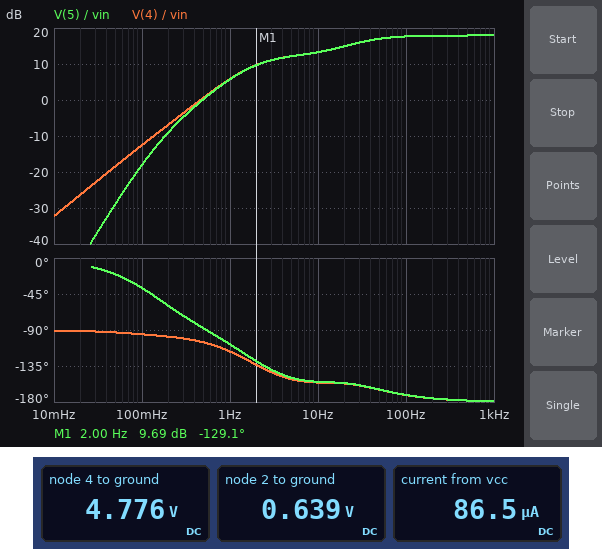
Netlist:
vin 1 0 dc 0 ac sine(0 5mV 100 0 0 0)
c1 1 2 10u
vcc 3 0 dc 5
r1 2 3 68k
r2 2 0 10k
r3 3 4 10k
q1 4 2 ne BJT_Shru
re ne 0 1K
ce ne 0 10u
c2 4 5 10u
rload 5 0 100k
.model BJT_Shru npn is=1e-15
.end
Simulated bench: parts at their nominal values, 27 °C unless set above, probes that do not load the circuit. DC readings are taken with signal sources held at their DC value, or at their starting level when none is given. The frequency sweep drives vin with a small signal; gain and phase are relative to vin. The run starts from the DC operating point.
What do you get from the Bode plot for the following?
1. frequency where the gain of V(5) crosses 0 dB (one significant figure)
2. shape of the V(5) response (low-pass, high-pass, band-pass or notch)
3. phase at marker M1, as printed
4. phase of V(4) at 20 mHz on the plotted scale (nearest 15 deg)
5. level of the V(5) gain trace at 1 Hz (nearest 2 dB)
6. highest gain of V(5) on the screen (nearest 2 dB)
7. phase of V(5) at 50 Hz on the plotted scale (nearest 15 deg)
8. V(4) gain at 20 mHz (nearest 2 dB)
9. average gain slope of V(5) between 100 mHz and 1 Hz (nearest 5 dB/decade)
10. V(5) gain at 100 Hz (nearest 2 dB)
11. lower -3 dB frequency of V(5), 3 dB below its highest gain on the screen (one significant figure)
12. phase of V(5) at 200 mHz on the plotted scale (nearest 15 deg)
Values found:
500 mHz
high-pass
-129.1 deg
-90 deg
6 dB
18 dB
-165 deg
-26 dB
25 dB/decade
18 dB
20 Hz
-60 deg
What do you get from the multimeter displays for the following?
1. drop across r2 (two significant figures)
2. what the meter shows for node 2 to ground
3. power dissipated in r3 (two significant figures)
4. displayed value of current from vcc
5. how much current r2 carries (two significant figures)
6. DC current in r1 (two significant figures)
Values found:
640 mV
0.639 V
5.0 µW
86.5 µA
64 µA
64 µA
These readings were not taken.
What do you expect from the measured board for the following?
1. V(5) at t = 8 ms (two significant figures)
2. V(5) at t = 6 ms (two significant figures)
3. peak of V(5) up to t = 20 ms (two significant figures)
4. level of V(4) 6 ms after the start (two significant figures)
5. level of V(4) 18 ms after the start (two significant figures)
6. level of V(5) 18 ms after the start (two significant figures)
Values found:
33 mV
27 mV
37 mV
4.8 V
4.8 V
33 mV
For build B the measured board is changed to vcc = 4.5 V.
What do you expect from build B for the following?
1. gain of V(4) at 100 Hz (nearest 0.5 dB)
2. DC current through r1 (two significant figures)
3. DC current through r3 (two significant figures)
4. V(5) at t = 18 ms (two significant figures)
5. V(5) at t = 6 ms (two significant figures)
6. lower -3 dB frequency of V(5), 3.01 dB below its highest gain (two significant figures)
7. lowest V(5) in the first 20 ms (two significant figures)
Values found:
3.0 dB
58 µA
4.1 µA
6.3 mV
4.4 mV
2.6 Hz
-7.7 mV
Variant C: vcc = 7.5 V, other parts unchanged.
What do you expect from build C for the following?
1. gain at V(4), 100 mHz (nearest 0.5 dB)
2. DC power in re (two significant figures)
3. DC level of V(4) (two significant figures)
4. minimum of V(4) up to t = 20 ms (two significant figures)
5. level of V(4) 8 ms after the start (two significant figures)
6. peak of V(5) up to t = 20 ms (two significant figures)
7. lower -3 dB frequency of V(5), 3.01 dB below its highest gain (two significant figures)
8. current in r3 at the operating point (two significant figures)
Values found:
-7.0 dB
67 µW
4.9 V
4.7 V
5.0 V
220 mV
180 Hz
260 µA
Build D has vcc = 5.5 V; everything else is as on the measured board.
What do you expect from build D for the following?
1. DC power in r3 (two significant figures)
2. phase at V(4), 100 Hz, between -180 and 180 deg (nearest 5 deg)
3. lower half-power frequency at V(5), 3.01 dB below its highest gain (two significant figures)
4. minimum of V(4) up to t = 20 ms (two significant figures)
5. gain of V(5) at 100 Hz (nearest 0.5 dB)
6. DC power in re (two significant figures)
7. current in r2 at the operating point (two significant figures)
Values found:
34 µW
-160 deg
47 Hz
4.8 V
25.5 dB
3.5 µW
70 µA
